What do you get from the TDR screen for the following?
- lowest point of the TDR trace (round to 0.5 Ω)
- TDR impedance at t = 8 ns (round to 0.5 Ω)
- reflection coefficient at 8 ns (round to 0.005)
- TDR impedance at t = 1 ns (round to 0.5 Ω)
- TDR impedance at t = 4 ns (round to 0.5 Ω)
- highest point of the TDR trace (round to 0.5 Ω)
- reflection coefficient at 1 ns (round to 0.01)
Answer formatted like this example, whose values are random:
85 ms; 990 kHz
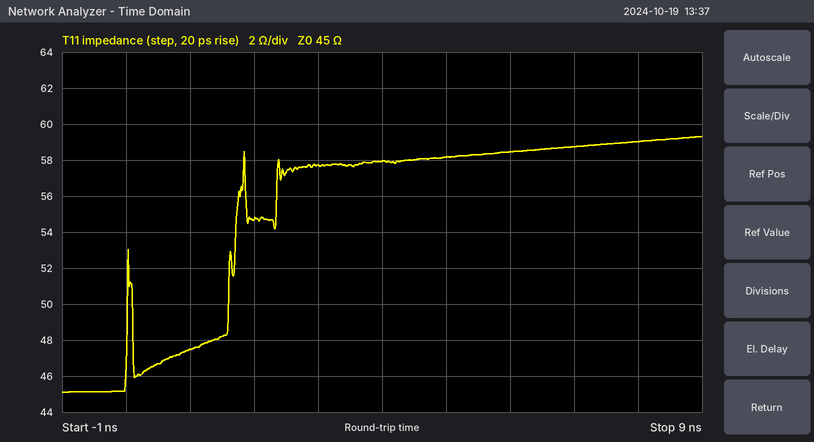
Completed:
45.0 Ω; 59.0 Ω; +0.135; 47.5 Ω; 58.0 Ω; 59.5 Ω; +0.03
